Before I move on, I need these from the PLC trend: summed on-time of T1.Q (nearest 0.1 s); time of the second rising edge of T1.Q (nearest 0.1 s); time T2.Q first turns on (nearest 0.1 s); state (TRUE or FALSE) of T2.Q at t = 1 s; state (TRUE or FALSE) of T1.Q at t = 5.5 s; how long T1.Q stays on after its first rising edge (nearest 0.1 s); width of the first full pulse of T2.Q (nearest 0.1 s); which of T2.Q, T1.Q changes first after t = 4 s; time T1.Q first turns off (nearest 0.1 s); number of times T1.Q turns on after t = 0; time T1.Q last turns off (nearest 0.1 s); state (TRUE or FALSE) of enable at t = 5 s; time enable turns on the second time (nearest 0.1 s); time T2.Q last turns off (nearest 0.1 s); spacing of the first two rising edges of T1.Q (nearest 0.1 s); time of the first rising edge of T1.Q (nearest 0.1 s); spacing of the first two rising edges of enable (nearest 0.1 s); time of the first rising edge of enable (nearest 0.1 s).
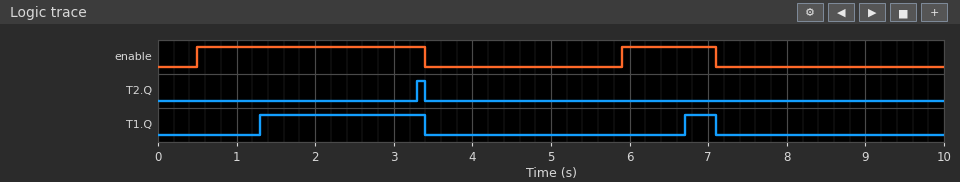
2.5 s
6.7 s
3.3 s
FALSE
FALSE
2.1 s
0.1 s
T1.Q
3.4 s
2
7.1 s
FALSE
5.9 s
3.4 s
5.4 s
1.3 s
5.4 s
0.5 s
